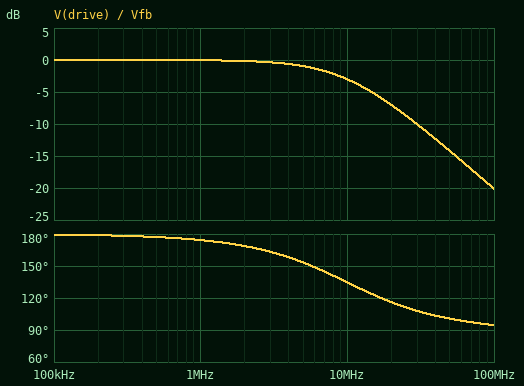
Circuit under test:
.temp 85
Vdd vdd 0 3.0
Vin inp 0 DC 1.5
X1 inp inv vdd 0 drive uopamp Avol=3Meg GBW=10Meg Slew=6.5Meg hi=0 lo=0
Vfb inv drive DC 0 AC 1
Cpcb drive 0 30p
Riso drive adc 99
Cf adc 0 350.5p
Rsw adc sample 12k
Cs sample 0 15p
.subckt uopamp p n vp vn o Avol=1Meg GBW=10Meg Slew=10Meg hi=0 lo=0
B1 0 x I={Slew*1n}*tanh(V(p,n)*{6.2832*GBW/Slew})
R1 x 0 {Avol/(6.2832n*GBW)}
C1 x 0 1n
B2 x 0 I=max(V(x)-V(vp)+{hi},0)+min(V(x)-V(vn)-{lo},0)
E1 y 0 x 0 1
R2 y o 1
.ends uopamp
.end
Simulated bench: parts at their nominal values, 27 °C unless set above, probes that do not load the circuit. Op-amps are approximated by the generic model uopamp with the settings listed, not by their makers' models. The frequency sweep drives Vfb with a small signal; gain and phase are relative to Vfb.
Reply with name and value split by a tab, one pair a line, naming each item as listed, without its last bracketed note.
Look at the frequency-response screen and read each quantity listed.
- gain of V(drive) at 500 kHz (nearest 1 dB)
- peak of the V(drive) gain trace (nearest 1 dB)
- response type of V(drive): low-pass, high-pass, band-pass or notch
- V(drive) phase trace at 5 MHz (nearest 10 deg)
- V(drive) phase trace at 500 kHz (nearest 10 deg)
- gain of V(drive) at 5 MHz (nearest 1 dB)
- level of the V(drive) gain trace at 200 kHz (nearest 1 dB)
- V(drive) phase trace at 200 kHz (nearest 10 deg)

gain of V(drive) at 500 kHz	0 dB
peak of the V(drive) gain trace	0 dB
response type of V(drive): low-pass, high-pass, band-pass or notch	low-pass
V(drive) phase trace at 5 MHz	150 deg
V(drive) phase trace at 500 kHz	180 deg
gain of V(drive) at 5 MHz	-1 dB
level of the V(drive) gain trace at 200 kHz	0 dB
V(drive) phase trace at 200 kHz	180 deg
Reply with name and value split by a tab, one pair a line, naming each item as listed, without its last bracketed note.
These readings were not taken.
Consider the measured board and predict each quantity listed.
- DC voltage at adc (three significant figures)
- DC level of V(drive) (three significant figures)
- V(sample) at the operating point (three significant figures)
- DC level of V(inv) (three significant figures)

DC voltage at adc	1.50 V
DC level of V(drive)	1.50 V
V(sample) at the operating point	1.50 V
DC level of V(inv)	1.50 V
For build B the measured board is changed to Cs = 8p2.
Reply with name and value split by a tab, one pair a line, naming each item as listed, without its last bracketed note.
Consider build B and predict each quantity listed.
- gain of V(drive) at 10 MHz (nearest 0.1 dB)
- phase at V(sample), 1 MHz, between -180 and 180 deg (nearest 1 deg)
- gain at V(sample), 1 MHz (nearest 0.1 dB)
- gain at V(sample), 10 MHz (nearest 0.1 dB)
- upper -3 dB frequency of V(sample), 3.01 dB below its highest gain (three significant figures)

gain of V(drive) at 10 MHz	-3.0 dB
phase at V(sample), 1 MHz, between -180 and 180 deg	130 deg
gain at V(sample), 1 MHz	-1.7 dB
gain at V(sample), 10 MHz	-26.6 dB
upper -3 dB frequency of V(sample), 3.01 dB below its highest gain	1.42 MHz
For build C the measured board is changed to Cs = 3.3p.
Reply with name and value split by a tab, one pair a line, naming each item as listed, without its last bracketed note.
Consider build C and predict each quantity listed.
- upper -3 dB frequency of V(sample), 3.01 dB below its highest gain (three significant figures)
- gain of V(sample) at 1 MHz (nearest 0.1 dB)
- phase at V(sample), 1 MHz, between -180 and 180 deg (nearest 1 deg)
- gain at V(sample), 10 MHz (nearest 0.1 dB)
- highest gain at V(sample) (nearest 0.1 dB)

upper -3 dB frequency of V(sample), 3.01 dB below its highest gain	2.59 MHz
gain of V(sample) at 1 MHz	-0.5 dB
phase at V(sample), 1 MHz, between -180 and 180 deg	148 deg
gain at V(sample), 10 MHz	-19.2 dB
highest gain at V(sample)	0 dB
